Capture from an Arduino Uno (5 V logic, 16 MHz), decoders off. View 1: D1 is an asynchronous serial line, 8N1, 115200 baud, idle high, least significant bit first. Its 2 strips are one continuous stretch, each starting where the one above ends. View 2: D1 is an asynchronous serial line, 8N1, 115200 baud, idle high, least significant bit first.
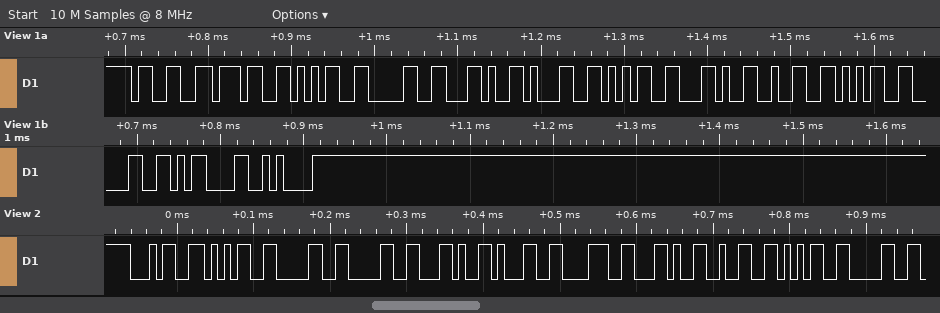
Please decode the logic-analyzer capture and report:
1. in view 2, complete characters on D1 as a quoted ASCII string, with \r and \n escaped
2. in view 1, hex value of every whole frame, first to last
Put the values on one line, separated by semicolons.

"4500,18,250"; 0x33 0x37 0x35 0x30 0x2C 0x31 0x35 0x2C 0x32 0x35 0x30 0x0D 0x0A
